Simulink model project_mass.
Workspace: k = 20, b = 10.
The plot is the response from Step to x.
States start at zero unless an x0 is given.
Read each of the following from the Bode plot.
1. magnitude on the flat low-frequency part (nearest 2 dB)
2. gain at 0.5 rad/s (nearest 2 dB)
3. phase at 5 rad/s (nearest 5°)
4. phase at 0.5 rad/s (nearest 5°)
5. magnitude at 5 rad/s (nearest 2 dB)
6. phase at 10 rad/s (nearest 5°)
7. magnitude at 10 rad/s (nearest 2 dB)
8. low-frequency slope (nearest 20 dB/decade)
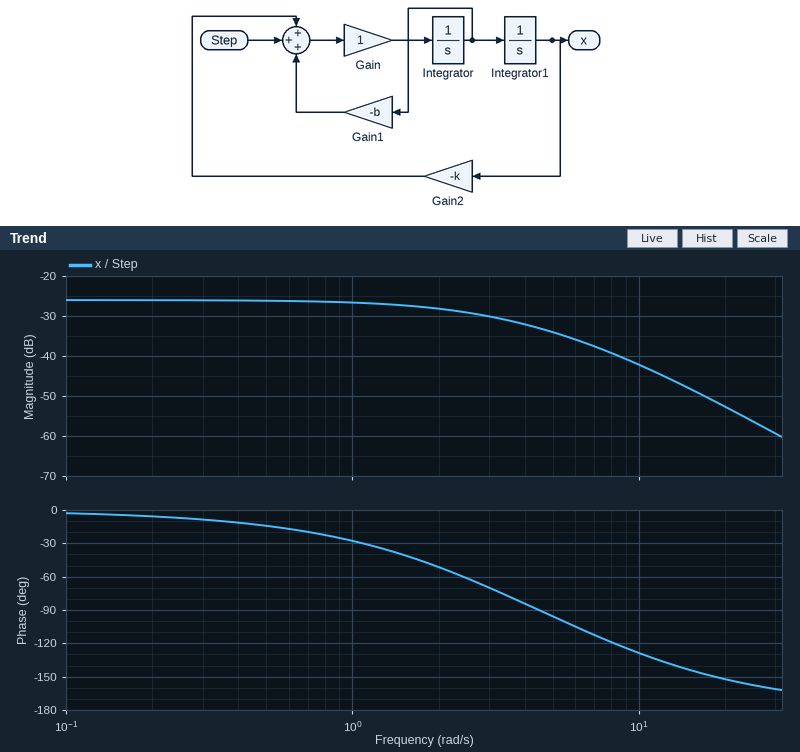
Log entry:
-26 dB
-26 dB
-95°
-15°
-34 dB
-130°
-42 dB
0 dB/decade
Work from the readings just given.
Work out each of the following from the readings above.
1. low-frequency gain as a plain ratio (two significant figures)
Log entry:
0.050
